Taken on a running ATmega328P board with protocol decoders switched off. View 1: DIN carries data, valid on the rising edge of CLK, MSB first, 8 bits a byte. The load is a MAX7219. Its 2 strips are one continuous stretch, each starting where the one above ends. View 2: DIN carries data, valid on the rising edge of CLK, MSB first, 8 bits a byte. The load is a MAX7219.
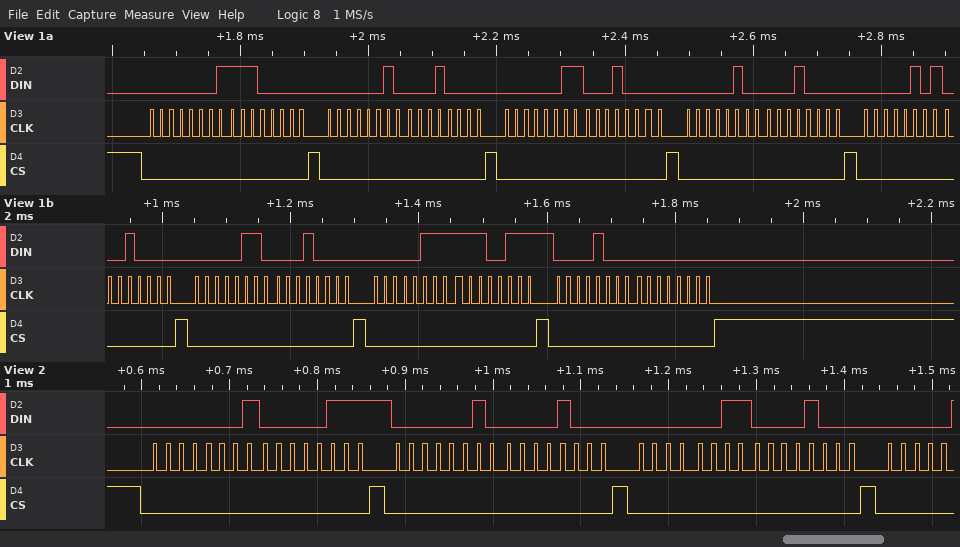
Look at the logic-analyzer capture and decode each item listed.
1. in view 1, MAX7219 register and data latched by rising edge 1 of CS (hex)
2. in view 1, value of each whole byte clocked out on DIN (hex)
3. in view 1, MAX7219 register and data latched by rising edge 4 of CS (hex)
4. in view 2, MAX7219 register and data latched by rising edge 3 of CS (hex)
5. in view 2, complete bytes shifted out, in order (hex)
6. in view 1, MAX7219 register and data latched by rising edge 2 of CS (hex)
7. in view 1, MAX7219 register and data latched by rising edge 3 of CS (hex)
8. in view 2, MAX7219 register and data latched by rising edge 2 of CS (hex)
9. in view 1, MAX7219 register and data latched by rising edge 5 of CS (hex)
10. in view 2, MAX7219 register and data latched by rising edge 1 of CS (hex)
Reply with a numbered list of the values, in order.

1. register 0x1, data 0xE0
2. 01 E0 02 10 03 10 04 10 05 10 06 10 07 E7 08 00
3. register 0x4, data 0x10
4. register 0x3, data 0x08
5. 01 07 02 08 03 08
6. register 0x2, data 0x10
7. register 0x3, data 0x10
8. register 0x2, data 0x08
9. register 0x5, data 0x10
10. register 0x1, data 0x07
